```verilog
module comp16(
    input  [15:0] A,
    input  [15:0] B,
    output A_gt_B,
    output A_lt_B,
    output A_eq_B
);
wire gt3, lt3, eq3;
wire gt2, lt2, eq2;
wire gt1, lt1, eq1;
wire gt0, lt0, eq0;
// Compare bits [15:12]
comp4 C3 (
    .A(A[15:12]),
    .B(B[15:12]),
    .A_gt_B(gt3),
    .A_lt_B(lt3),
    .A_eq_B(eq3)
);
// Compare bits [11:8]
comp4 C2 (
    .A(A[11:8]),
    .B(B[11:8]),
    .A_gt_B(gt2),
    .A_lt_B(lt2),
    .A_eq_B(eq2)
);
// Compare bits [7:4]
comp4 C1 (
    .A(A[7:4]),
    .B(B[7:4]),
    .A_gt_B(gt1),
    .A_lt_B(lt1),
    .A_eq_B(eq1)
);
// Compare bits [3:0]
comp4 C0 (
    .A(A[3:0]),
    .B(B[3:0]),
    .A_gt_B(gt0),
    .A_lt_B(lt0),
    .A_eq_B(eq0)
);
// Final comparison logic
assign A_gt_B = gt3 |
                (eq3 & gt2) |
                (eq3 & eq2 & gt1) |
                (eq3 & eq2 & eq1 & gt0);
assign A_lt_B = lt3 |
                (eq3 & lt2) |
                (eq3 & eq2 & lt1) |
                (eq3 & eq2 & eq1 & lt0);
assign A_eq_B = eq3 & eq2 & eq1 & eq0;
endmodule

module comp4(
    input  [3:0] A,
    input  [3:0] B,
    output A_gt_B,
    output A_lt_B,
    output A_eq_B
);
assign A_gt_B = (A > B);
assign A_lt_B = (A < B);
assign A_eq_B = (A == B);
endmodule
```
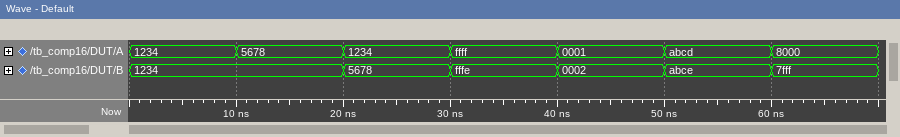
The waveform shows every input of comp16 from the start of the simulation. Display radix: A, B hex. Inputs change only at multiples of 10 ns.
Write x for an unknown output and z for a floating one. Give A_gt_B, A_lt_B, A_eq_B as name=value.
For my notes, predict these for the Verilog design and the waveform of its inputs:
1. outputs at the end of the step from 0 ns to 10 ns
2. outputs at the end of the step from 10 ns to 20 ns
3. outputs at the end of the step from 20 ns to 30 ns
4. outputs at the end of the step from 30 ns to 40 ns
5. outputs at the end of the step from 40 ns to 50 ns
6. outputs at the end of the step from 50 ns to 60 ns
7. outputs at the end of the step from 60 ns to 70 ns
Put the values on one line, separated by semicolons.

A_gt_B=0, A_lt_B=0, A_eq_B=1; A_gt_B=1, A_lt_B=0, A_eq_B=0; A_gt_B=0, A_lt_B=1, A_eq_B=0; A_gt_B=1, A_lt_B=0, A_eq_B=0; A_gt_B=0, A_lt_B=1, A_eq_B=0; A_gt_B=0, A_lt_B=1, A_eq_B=0; A_gt_B=1, A_lt_B=0, A_eq_B=0
